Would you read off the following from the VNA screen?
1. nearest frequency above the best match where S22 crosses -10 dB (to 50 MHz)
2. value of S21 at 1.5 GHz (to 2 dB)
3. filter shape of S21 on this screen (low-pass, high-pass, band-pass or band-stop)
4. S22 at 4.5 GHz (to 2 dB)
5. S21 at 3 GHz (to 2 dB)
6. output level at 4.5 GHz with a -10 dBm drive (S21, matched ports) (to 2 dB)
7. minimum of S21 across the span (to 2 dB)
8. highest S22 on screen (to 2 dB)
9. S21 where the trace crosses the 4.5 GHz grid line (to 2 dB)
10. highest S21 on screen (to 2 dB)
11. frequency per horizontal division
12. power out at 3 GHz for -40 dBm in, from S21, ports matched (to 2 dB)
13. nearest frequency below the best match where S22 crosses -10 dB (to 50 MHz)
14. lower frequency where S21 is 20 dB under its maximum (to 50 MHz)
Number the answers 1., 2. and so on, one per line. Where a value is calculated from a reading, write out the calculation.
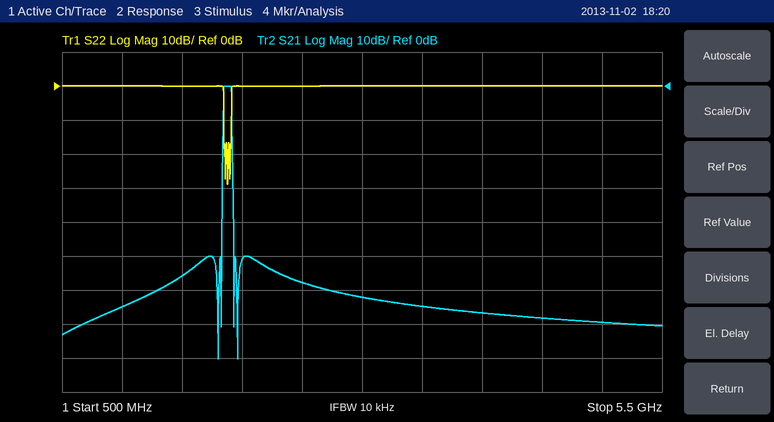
1. 1.90 GHz
2. -56 dB
3. band-pass
4. 0 dB
5. -62 dB
6. -10 dBm + (-68 dB) = -78 dBm
7. -80 dB
8. 0 dB
9. -68 dB
10. 0 dB
11. 500 MHz
12. -40 dBm + (-62 dB) = -102 dBm
13. 1.85 GHz
14. 1.85 GHz
